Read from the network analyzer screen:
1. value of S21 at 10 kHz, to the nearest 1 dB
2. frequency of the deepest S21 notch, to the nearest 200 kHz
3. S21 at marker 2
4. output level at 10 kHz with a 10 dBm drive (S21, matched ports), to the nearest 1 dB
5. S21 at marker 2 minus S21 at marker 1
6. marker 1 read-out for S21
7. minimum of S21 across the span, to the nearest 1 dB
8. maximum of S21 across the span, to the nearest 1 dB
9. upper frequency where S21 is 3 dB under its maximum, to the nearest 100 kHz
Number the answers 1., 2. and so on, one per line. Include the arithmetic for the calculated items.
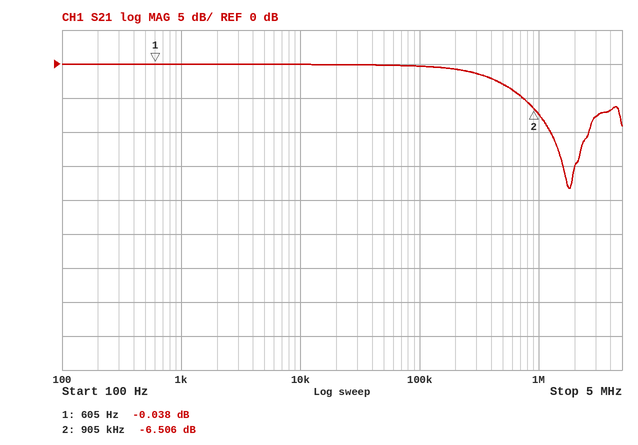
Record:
1. 0 dB
2. 1.8 MHz
3. -6.506 dB
4. 10 dBm + (0 dB) = 10 dBm
5. -6.506 − (-0.038) = -6.468 dB
6. -0.038 dB
7. -18 dB
8. 0 dB
9. 500 kHz
